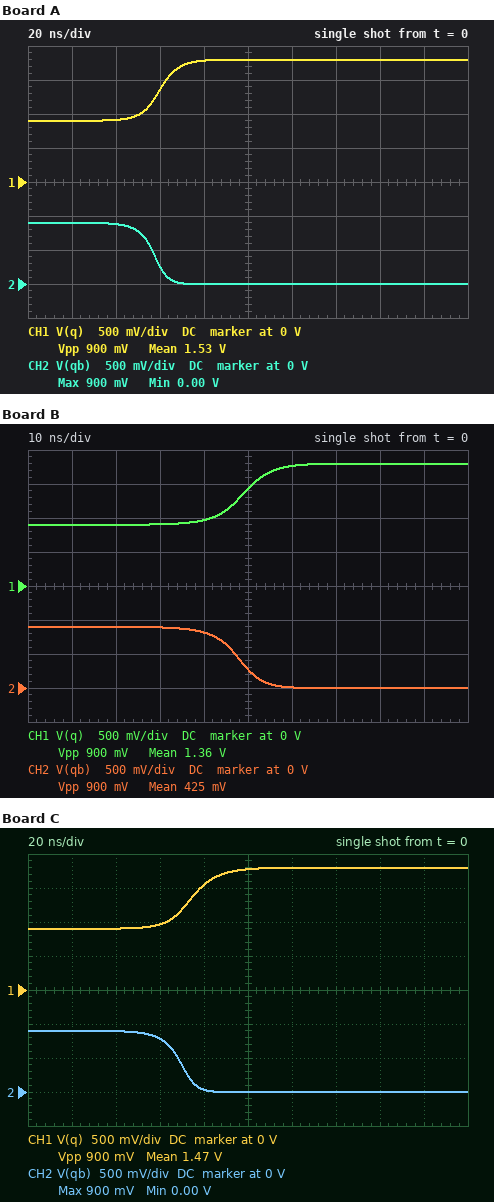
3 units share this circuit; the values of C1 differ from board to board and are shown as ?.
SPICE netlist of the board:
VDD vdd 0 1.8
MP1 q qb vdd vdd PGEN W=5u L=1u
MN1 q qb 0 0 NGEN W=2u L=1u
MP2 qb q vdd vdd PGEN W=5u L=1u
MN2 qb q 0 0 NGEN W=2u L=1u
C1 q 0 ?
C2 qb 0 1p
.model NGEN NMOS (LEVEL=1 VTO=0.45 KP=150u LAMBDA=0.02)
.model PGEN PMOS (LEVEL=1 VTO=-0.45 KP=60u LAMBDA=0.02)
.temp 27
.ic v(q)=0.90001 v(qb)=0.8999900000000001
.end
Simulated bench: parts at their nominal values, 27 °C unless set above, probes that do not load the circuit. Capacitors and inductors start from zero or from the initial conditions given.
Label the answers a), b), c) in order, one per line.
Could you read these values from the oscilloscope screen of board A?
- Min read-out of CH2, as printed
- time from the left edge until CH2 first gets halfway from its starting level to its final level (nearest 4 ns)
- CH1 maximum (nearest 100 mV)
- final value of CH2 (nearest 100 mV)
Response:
a) 0.00 V
b) 56 ns
c) 1.8 V
d) 0 V
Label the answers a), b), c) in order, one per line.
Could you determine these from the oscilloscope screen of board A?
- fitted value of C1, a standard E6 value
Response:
a) 2.2 pF
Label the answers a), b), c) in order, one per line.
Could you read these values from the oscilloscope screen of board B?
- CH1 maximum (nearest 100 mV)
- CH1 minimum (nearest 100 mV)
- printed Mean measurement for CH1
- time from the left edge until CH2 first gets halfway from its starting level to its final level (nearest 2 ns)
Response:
a) 1.8 V
b) 900 mV
c) 1.36 V
d) 48 ns
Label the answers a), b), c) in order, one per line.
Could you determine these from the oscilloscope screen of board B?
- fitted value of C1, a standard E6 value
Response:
a) 1.5 pF
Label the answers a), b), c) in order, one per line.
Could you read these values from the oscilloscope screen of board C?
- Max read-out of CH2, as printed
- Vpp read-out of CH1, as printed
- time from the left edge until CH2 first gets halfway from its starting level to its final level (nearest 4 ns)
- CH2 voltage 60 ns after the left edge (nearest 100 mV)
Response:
a) 900 mV
b) 900 mV
c) 68 ns
d) 800 mV
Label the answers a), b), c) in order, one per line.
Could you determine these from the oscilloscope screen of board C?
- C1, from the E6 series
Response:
a) 3.3 pF
